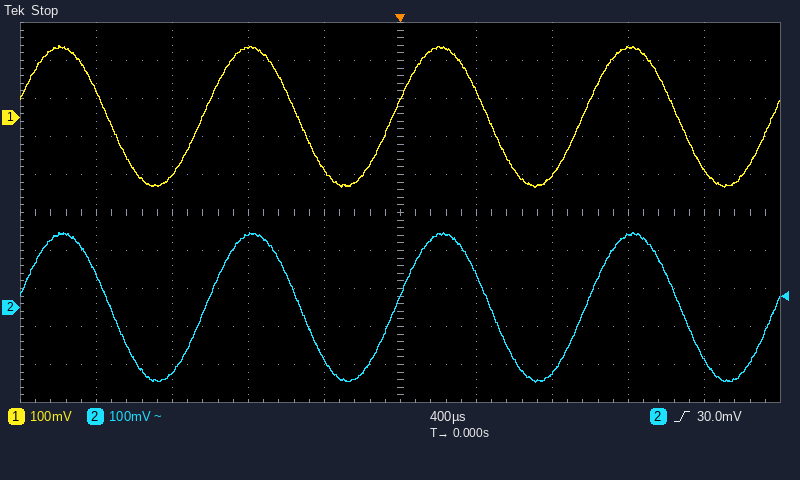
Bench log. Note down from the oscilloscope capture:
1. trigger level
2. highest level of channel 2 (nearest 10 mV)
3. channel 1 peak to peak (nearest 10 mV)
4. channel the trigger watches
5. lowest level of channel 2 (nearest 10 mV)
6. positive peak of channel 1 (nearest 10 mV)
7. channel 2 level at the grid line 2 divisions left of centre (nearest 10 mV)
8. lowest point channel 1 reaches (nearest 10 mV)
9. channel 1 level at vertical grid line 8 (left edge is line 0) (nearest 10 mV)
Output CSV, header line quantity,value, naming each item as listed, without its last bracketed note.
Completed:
quantity,value
trigger level,30.0 mV
highest level of channel 2,200 mV
channel 1 peak to peak,370 mV
channel the trigger watches,channel 2
lowest level of channel 2,-200 mV
positive peak of channel 1,190 mV
channel 2 level at the grid line 2 divisions left of centre,190 mV
lowest point channel 1 reaches,-180 mV
channel 1 level at vertical grid line 8 (left edge is line 0),180 mV
